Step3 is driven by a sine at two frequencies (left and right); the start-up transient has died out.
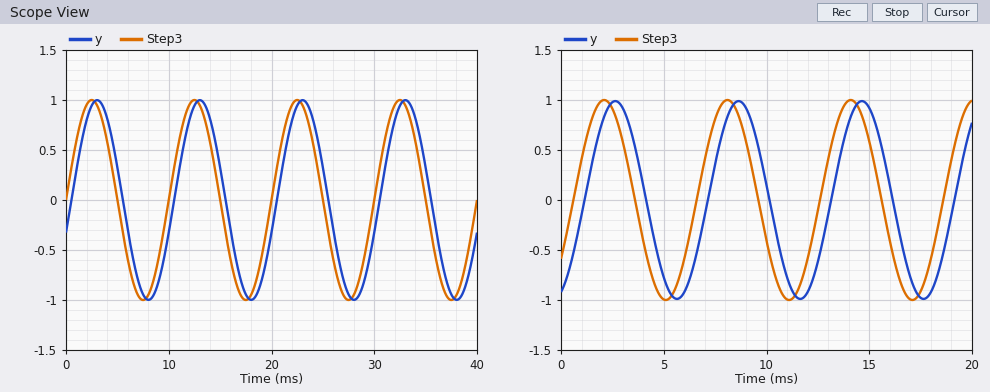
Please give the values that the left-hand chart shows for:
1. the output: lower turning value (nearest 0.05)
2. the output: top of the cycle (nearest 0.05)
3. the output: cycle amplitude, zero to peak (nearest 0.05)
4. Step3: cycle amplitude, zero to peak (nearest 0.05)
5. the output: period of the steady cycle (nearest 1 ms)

-1.00
1.00
1.00
1.00
10 ms
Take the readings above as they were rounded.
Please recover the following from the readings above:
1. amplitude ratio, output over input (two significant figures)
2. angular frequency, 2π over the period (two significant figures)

1.0
0.63 rad/ms
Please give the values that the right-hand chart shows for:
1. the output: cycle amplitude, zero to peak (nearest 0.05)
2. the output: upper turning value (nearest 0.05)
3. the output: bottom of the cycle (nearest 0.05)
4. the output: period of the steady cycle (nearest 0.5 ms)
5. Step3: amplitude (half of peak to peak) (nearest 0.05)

1.00
1.00
-1.00
6.0 ms
1.00
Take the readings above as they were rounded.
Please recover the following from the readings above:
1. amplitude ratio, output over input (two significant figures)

1.0
